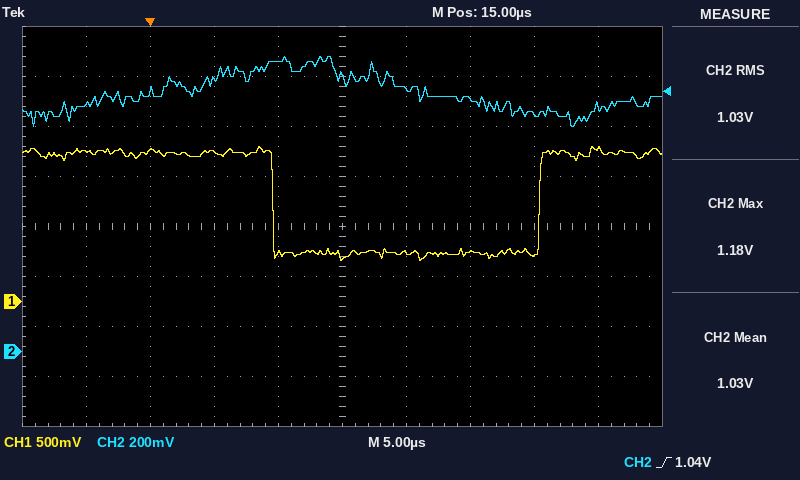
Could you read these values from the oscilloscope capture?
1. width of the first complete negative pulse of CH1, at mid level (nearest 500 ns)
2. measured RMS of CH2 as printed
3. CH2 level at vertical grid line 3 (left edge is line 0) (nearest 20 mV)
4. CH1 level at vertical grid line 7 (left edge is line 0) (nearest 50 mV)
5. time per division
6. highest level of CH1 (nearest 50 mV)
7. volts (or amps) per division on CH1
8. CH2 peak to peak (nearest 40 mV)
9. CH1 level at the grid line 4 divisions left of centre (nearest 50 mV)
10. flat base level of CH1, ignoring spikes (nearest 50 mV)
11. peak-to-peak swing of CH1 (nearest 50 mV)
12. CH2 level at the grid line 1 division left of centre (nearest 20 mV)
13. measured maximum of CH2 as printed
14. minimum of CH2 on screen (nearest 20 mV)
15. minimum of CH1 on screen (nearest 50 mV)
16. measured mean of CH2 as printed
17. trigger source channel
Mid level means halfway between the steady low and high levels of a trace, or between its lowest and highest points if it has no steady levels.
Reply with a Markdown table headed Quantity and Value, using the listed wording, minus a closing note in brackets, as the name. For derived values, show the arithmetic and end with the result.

| Quantity | Value |
|---|---|
| width of the first complete negative pulse of CH1, at mid level | 21.0 µs |
| measured RMS of CH2 as printed | 1.03 V |
| CH2 level at vertical grid line 3 (left edge is line 0) | 1.08 V |
| CH1 level at vertical grid line 7 (left edge is line 0) | 500 mV |
| time per division | 5 µs |
| highest level of CH1 | 1.55 V |
| volts (or amps) per division on CH1 | 500 mV |
| CH2 peak to peak | 280 mV |
| CH1 level at the grid line 4 divisions left of centre | 1.50 V |
| flat base level of CH1, ignoring spikes | 500 mV |
| peak-to-peak swing of CH1 | 1.55 V − (400 mV) = 1.15 V |
| CH2 level at the grid line 1 division left of centre | 1.16 V |
| measured maximum of CH2 as printed | 1.18 V |
| minimum of CH2 on screen | 900 mV |
| minimum of CH1 on screen | 400 mV |
| measured mean of CH2 as printed | 1.03 V |
| trigger source channel | CH2 |
